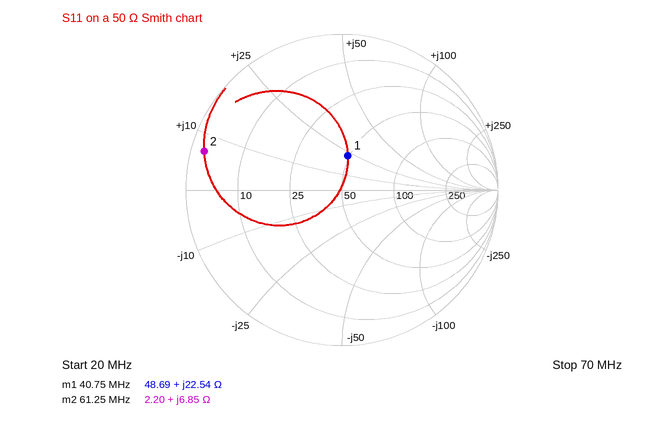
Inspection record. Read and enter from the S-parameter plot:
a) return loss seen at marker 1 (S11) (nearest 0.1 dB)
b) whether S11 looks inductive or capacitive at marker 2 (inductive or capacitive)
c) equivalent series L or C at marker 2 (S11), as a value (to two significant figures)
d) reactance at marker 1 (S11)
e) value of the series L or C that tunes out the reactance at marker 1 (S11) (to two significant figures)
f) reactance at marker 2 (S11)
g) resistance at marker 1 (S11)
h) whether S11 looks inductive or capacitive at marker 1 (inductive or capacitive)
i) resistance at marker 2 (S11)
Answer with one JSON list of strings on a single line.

["13.0 dB", "inductive", "18 nH", "+22.54 Ω", "170 pF", "+6.85 Ω", "48.69 Ω", "inductive", "2.20 Ω"]
